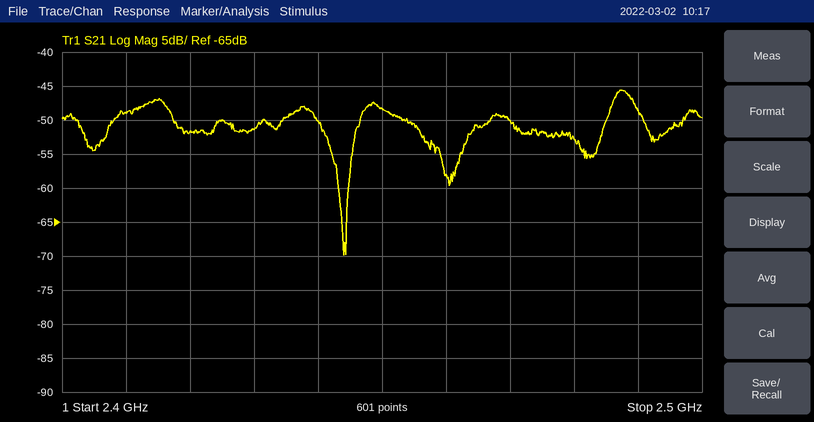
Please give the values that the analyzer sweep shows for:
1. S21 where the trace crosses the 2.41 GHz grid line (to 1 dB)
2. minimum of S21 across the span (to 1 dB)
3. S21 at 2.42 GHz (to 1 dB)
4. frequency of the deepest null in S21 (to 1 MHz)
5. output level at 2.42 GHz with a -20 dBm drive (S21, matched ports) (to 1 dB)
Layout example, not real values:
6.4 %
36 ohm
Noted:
-49 dB
-70 dB
-52 dB
2.444 GHz
-72 dBm
